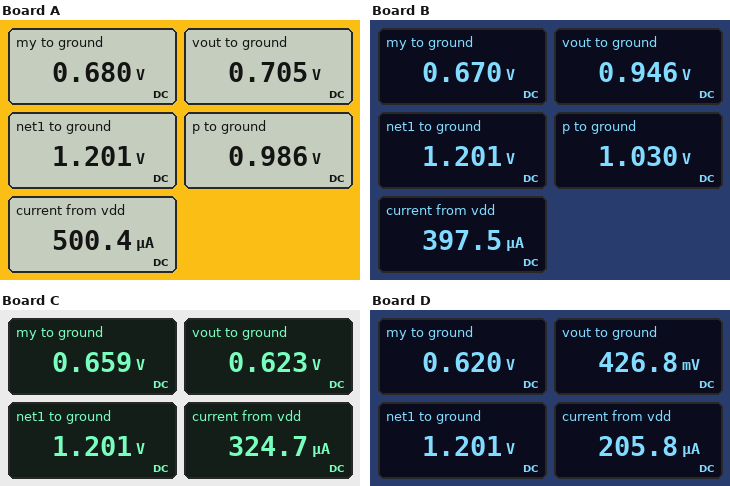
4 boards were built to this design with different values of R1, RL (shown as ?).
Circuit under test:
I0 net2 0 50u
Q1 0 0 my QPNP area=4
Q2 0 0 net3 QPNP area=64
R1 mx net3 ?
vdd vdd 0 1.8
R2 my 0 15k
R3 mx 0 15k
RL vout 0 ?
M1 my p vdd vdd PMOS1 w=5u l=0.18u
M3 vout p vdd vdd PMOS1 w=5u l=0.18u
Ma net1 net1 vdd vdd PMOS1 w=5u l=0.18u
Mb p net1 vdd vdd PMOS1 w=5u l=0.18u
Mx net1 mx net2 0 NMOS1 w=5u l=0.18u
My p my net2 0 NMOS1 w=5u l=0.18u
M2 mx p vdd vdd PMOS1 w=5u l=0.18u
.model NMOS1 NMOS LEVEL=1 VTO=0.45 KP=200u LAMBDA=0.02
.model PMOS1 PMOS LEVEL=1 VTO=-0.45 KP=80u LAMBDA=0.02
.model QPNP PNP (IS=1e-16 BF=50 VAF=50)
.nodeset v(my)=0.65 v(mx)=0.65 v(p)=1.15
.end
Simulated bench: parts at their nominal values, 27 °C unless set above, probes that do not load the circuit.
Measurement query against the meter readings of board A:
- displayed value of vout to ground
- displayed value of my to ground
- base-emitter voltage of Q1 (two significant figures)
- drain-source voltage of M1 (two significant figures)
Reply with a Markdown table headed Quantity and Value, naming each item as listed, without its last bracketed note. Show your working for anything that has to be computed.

| Quantity | Value |
|---|---|
| displayed value of vout to ground | 0.705 V |
| displayed value of my to ground | 0.680 V |
| base-emitter voltage of Q1 | 0 V - 680 mV = -680 mV |
| drain-source voltage of M1 | 680 mV - 1.8 V = -1.1 V |
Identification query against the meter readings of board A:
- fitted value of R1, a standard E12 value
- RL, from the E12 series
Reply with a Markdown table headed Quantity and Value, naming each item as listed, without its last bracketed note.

| Quantity | Value |
|---|---|
| fitted value of R1, a standard E12 value | 680 Ω |
| RL, from the E12 series | 4.7 kΩ |
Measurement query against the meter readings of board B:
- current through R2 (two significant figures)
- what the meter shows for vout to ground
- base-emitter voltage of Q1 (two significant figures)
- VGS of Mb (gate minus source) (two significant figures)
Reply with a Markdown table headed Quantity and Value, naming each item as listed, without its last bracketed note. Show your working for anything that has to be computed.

| Quantity | Value |
|---|---|
| current through R2 | (670 mV) / 15 kΩ = 45 µA |
| what the meter shows for vout to ground | 0.946 V |
| base-emitter voltage of Q1 | 0 V - 670 mV = -670 mV |
| VGS of Mb (gate minus source) | 1.201 V - 1.8 V = -600 mV |
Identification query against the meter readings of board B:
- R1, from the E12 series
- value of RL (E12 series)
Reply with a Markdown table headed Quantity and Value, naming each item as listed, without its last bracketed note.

| Quantity | Value |
|---|---|
| R1, from the E12 series | 1 kΩ |
| value of RL | 8.2 kΩ |
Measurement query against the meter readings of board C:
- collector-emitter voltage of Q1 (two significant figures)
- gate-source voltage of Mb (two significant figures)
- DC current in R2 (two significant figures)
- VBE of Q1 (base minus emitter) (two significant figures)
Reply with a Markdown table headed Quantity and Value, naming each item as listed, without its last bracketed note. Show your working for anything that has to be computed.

| Quantity | Value |
|---|---|
| collector-emitter voltage of Q1 | 0 V - 659 mV = -660 mV |
| gate-source voltage of Mb | 1.201 V - 1.8 V = -600 mV |
| DC current in R2 | (659 mV) / 15 kΩ = 44 µA |
| VBE of Q1 (base minus emitter) | 0 V - 659 mV = -660 mV |
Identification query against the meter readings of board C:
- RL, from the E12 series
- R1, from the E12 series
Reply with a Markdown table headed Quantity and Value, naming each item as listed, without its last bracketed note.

| Quantity | Value |
|---|---|
| RL, from the E12 series | 6.8 kΩ |
| R1, from the E12 series | 1.5 kΩ |
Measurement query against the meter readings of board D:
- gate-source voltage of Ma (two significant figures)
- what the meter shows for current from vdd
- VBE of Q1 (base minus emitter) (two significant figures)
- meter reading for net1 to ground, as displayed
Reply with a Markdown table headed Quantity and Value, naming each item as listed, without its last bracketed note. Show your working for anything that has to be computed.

| Quantity | Value |
|---|---|
| gate-source voltage of Ma | 1.201 V - 1.8 V = -600 mV |
| what the meter shows for current from vdd | 205.8 µA |
| VBE of Q1 (base minus emitter) | 0 V - 620 mV = -620 mV |
| meter reading for net1 to ground, as displayed | 1.201 V |
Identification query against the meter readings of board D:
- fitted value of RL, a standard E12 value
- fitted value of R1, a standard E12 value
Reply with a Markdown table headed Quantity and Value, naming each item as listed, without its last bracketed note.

| Quantity | Value |
|---|---|
| fitted value of RL, a standard E12 value | 8.2 kΩ |
| fitted value of R1, a standard E12 value | 6.8 kΩ |
